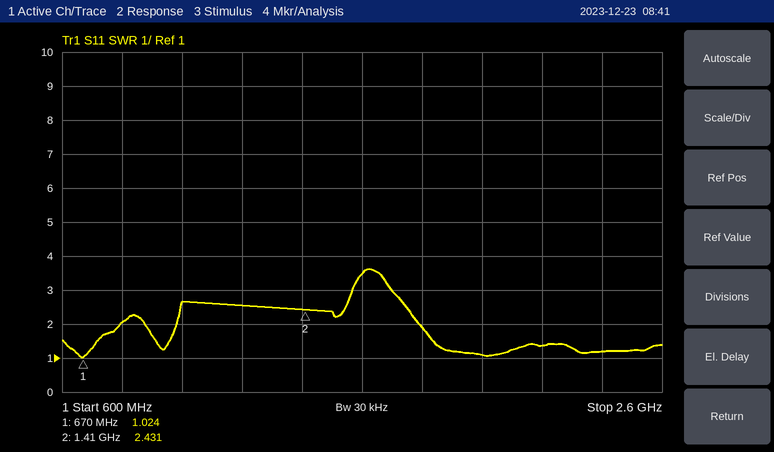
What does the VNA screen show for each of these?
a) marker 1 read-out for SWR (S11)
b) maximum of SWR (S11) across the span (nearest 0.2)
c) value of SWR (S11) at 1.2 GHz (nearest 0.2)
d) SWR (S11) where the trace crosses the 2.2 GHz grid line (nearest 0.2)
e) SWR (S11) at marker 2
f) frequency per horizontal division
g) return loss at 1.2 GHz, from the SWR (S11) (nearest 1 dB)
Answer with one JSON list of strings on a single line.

["1.024", "3.6", "2.6", "1.4", "2.431", "200 MHz", "7 dB"]
